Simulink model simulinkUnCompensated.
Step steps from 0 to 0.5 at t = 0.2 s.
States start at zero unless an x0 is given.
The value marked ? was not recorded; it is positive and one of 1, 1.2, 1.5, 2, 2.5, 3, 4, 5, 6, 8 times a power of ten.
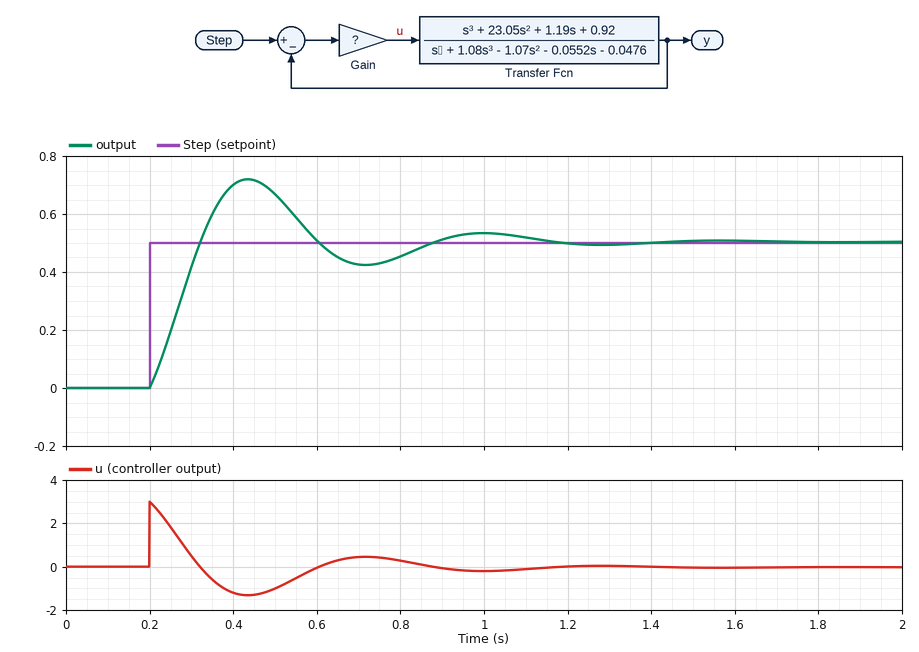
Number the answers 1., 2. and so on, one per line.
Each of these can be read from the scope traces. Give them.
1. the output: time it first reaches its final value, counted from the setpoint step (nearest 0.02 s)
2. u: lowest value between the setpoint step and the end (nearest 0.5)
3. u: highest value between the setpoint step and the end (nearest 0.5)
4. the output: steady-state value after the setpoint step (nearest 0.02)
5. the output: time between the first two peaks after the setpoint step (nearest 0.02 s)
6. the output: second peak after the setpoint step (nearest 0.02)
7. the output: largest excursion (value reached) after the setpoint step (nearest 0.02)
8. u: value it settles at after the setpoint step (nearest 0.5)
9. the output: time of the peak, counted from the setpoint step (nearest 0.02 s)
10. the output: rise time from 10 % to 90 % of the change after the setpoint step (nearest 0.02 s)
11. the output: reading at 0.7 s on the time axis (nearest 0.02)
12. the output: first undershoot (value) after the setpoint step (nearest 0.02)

1. 0.12 s
2. -1.5
3. 3.0
4. 0.50
5. 0.56 s
6. 0.54
7. 0.72
8. 0.0
9. 0.24 s
10. 0.10 s
11. 0.42
12. 0.42
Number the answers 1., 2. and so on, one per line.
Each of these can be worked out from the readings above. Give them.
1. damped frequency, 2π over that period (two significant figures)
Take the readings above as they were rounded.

1. 11 rad/s
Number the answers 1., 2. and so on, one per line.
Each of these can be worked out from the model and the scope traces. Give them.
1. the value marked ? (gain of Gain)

1. 6
